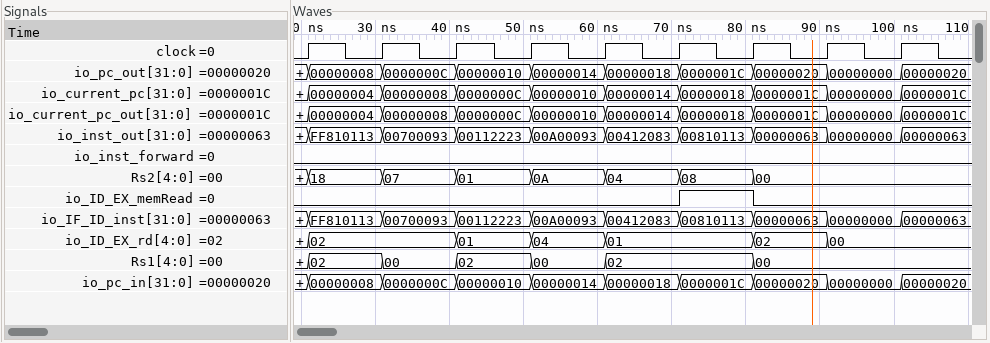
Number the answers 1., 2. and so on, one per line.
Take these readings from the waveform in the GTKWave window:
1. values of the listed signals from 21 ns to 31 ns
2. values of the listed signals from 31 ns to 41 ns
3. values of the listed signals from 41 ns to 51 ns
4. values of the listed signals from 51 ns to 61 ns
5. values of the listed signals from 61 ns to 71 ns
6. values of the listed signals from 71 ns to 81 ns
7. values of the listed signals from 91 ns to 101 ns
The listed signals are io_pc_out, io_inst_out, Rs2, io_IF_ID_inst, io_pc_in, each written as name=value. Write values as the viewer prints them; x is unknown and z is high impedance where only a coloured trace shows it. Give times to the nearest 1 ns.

1. io_pc_out=00000008, io_inst_out=FF810113, Rs2=18, io_IF_ID_inst=FF810113, io_pc_in=00000008
2. io_pc_out=0000000C, io_inst_out=00700093, Rs2=07, io_IF_ID_inst=00700093, io_pc_in=0000000C
3. io_pc_out=00000010, io_inst_out=00112223, Rs2=01, io_IF_ID_inst=00112223, io_pc_in=00000010
4. io_pc_out=00000014, io_inst_out=00A00093, Rs2=0A, io_IF_ID_inst=00A00093, io_pc_in=00000014
5. io_pc_out=00000018, io_inst_out=00412083, Rs2=04, io_IF_ID_inst=00412083, io_pc_in=00000018
6. io_pc_out=0000001C, io_inst_out=00810113, Rs2=08, io_IF_ID_inst=00810113, io_pc_in=0000001C
7. io_pc_out=00000000, io_inst_out=00000000, Rs2=00, io_IF_ID_inst=00000000, io_pc_in=00000000
